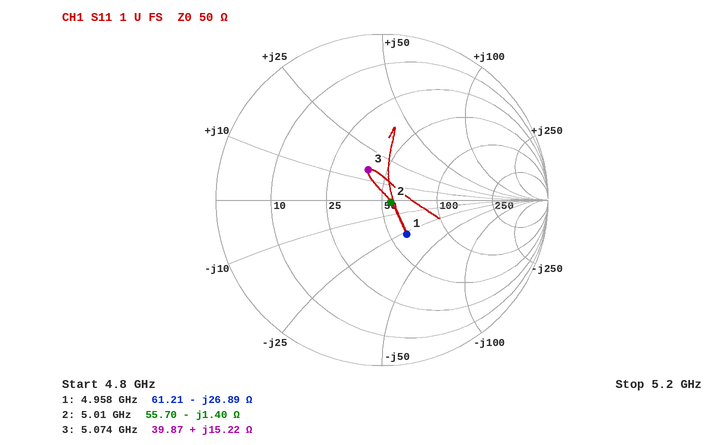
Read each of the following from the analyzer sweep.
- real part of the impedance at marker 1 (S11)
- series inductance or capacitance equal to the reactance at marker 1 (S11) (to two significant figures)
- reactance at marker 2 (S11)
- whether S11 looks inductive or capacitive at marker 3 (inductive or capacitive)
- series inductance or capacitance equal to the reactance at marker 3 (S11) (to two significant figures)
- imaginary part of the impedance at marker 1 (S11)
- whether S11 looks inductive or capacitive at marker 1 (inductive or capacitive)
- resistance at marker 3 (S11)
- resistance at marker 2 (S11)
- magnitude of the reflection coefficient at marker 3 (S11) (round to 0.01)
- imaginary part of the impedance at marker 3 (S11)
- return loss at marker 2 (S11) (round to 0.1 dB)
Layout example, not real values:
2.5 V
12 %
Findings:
61.21 Ω
1.2 pF
-1.40 Ω
inductive
480 pH
-26.89 Ω
capacitive
39.87 Ω
55.70 Ω
0.20
+15.22 Ω
25.1 dB
